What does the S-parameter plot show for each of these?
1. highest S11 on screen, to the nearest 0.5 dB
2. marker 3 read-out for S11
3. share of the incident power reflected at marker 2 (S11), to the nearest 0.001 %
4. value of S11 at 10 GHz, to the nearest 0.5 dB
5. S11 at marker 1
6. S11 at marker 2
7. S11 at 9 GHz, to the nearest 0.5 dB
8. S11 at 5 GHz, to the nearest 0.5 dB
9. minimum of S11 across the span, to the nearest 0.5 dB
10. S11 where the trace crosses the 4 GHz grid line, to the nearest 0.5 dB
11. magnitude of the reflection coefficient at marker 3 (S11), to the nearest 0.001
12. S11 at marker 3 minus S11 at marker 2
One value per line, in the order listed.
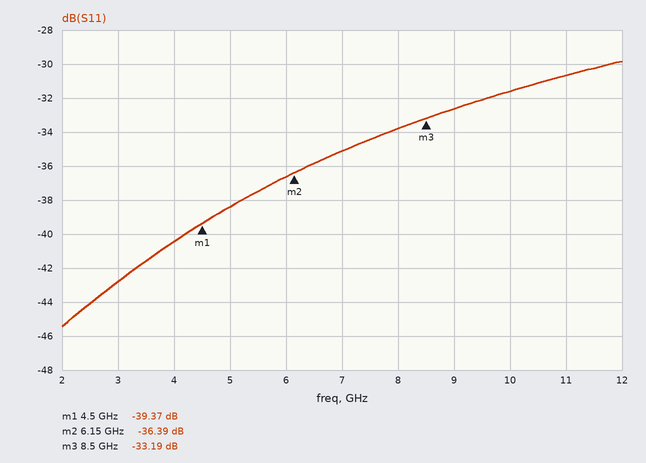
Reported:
-30.0 dB
-33.19 dB
0.023 %
-31.5 dB
-39.37 dB
-36.39 dB
-32.5 dB
-38.5 dB
-45.5 dB
-40.5 dB
0.022
3.20 dB
